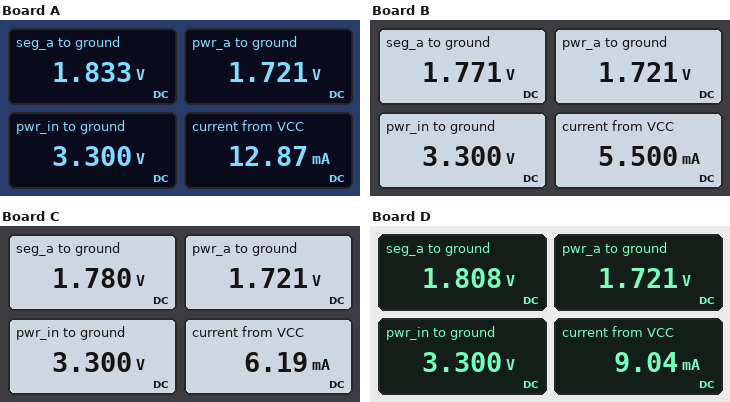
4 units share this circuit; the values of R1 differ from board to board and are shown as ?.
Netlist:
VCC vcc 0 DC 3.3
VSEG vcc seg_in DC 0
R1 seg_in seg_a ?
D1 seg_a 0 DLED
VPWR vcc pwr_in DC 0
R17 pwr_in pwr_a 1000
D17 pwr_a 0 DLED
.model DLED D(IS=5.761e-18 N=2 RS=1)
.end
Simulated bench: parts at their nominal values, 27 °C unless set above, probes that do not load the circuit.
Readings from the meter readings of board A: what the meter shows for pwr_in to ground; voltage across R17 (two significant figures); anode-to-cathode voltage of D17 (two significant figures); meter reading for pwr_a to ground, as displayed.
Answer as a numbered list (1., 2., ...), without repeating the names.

1. 3.300 V
2. 1.6 V
3. 1.7 V
4. 1.721 V
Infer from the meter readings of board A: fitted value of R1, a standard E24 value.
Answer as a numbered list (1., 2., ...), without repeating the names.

1. 130 Ω
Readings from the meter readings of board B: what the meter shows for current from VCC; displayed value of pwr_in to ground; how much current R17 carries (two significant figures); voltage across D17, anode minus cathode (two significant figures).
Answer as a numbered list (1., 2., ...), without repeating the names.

1. 5.500 mA
2. 3.300 V
3. 1.6 mA
4. 1.7 V
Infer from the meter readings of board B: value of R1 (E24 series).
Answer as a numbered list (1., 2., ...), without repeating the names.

1. 390 Ω
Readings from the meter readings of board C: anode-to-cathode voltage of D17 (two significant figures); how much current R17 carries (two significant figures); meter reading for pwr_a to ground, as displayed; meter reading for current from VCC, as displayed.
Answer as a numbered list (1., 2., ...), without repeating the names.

1. 1.7 V
2. 1.6 mA
3. 1.721 V
4. 6.19 mA
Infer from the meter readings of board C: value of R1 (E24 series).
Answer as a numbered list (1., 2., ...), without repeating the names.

1. 330 Ω
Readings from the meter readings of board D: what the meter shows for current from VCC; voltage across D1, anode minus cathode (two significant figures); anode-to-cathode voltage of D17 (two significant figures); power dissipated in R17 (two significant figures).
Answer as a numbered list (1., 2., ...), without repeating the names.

1. 9.04 mA
2. 1.8 V
3. 1.7 V
4. 2.5 mW
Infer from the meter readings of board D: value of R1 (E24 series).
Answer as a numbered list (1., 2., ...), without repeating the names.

1. 200 Ω
